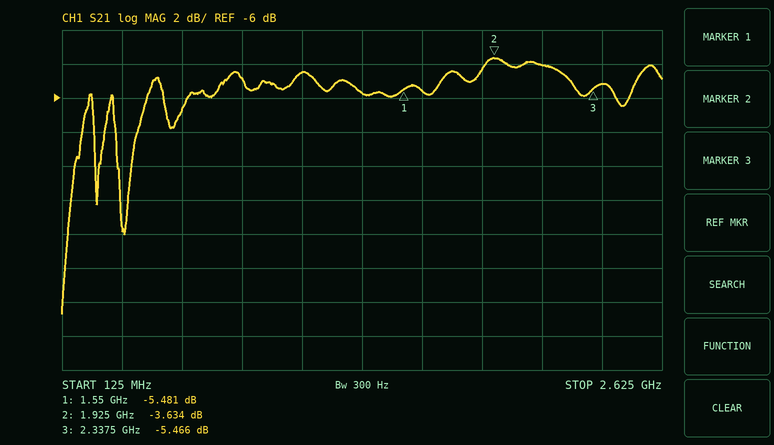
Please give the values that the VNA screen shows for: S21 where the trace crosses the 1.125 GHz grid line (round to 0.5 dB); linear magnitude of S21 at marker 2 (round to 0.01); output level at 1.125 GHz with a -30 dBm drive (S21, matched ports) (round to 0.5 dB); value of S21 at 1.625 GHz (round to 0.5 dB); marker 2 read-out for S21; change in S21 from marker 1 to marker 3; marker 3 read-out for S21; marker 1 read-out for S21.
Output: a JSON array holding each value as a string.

["-4.5 dB", "0.66", "-34.5 dBm", "-5.5 dB", "-3.634 dB", "0.015 dB", "-5.466 dB", "-5.481 dB"]
